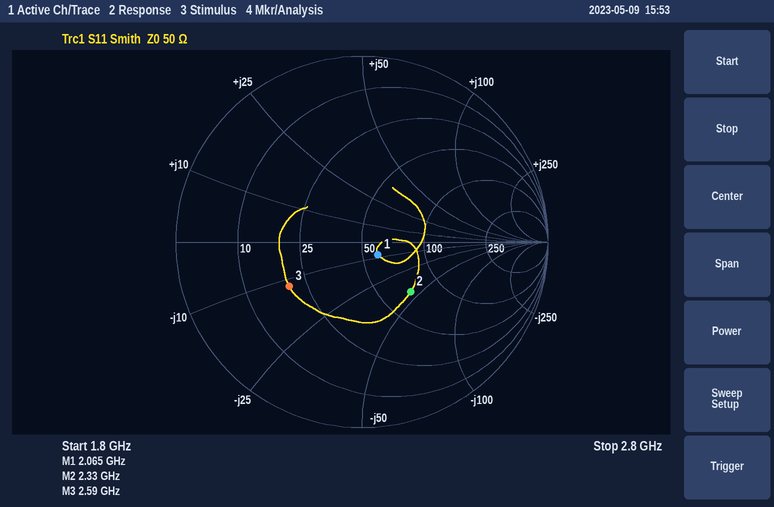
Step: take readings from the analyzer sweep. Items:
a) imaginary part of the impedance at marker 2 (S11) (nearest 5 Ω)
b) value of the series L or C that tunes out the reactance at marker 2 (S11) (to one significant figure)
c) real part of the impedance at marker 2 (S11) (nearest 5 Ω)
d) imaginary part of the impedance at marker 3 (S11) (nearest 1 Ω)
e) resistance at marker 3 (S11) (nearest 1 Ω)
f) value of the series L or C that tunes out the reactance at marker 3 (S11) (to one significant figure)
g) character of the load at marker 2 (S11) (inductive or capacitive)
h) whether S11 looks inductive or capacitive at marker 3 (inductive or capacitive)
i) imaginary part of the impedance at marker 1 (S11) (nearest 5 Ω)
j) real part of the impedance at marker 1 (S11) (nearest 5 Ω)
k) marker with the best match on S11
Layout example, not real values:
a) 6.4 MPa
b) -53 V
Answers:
a) -45 Ω
b) 3 nH
c) 70 Ω
d) -12 Ω
e) 20 Ω
f) 700 pH
g) capacitive
h) capacitive
i) -10 Ω
j) 60 Ω
k) marker 1
